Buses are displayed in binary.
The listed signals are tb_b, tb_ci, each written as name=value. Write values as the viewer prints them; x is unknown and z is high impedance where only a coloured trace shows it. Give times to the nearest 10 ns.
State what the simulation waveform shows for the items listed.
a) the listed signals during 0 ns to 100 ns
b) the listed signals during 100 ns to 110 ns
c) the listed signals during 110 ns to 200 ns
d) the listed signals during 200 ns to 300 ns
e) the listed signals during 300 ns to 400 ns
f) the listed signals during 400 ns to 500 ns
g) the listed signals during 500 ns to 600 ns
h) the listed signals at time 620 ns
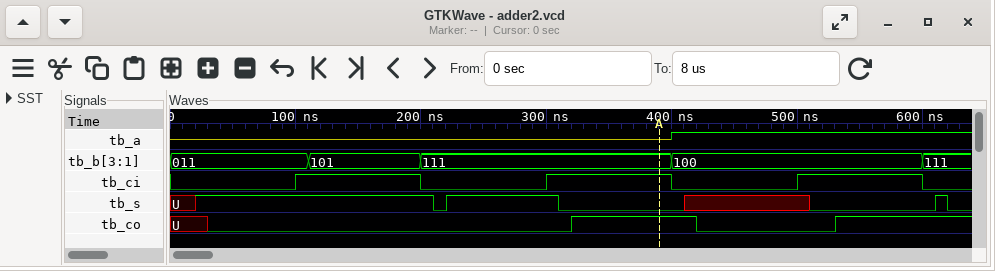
tb_b=011, tb_ci=0
tb_b=011, tb_ci=1
tb_b=101, tb_ci=1
tb_b=111, tb_ci=0
tb_b=111, tb_ci=1
tb_b=100, tb_ci=0
tb_b=100, tb_ci=1
tb_b=111, tb_ci=0
